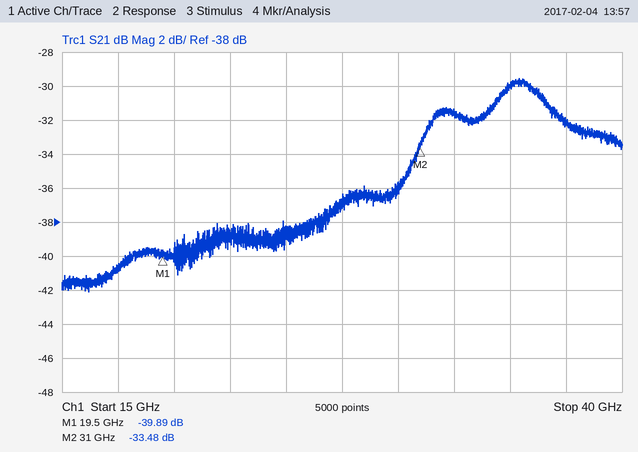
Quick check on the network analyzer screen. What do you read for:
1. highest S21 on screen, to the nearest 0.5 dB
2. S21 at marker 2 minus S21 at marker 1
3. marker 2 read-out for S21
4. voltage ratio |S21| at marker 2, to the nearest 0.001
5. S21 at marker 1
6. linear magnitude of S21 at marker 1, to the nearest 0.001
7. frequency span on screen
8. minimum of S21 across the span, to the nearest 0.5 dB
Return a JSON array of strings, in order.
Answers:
["-29.5 dB", "6.41 dB", "-33.48 dB", "0.021", "-39.89 dB", "0.010", "25 GHz", "-42.0 dB"]
